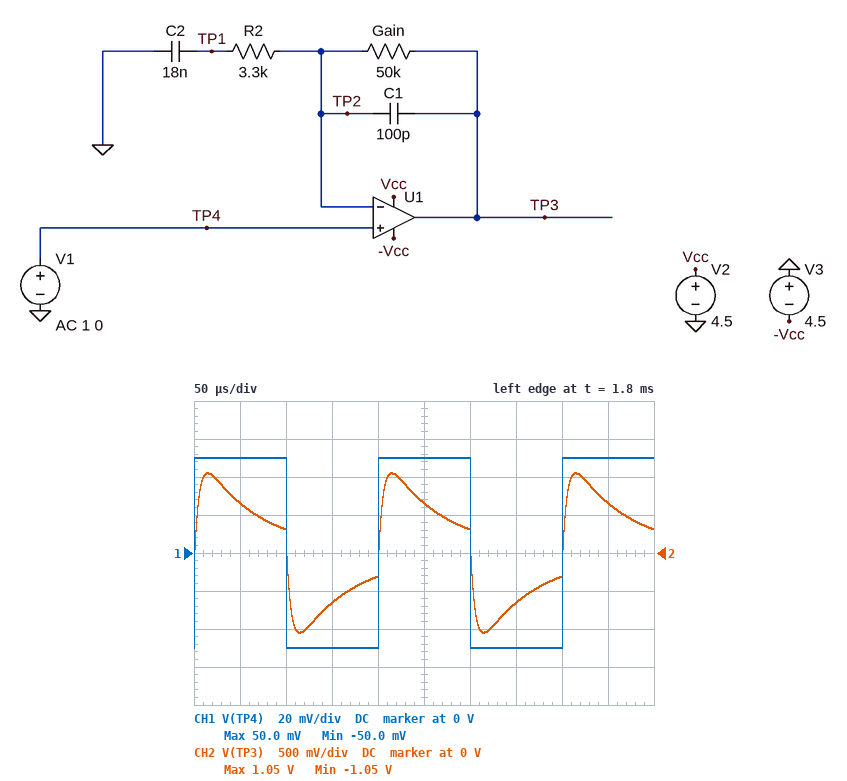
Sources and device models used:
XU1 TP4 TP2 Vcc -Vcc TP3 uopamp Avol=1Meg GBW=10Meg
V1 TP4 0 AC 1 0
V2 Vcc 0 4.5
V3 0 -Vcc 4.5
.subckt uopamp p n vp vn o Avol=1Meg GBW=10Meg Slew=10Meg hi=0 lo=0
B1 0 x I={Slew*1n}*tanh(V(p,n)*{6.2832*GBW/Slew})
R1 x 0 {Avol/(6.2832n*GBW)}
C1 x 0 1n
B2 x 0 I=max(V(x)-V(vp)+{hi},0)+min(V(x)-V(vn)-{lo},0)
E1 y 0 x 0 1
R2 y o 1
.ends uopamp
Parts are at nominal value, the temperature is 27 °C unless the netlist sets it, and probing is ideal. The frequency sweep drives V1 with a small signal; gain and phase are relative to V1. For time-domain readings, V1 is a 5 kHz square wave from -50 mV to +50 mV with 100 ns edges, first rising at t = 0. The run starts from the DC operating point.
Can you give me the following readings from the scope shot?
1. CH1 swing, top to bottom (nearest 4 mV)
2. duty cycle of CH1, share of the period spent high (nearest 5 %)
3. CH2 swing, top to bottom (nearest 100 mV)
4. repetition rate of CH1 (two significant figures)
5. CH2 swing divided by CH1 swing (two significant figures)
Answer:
100 mV
50 %
2.1 V
5.0 kHz
21
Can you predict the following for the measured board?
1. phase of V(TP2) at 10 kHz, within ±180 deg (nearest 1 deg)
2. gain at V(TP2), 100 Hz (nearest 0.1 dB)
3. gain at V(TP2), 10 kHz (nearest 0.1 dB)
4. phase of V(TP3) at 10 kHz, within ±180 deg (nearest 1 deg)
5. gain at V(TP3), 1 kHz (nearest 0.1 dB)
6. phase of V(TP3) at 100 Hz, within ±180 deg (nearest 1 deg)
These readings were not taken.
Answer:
-1 deg
0 dB
0 dB
-3 deg
15.2 dB
29 deg
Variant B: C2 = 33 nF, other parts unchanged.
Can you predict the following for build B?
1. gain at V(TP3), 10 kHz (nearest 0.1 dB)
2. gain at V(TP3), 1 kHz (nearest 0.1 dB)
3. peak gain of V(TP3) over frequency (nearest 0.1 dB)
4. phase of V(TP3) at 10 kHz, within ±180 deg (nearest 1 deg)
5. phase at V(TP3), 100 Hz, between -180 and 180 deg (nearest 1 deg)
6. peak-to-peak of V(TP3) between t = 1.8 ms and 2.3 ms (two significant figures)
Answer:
23.7 dB
19.3 dB
23.8 dB
-9 deg
44 deg
1.9 V
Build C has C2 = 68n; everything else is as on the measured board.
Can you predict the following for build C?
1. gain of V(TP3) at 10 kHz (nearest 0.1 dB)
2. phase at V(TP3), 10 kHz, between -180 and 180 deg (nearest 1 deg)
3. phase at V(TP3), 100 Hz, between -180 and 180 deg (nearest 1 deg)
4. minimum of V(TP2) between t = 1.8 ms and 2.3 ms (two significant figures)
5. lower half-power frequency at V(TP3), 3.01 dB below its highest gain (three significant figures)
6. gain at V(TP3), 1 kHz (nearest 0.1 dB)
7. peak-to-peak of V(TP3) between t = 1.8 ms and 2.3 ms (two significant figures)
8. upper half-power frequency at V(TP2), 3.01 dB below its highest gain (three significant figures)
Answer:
23.7 dB
-13 deg
58 deg
-50 mV
676 Hz
22.4 dB
1.8 V
9.47 MHz
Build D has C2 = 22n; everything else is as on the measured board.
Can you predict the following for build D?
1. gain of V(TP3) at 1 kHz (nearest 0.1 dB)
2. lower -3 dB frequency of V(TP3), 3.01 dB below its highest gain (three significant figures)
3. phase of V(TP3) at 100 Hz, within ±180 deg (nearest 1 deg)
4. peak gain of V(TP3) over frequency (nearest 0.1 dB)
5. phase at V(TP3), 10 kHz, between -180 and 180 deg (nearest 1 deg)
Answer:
16.6 dB
1.93 kHz
34 deg
23.6 dB
-6 deg
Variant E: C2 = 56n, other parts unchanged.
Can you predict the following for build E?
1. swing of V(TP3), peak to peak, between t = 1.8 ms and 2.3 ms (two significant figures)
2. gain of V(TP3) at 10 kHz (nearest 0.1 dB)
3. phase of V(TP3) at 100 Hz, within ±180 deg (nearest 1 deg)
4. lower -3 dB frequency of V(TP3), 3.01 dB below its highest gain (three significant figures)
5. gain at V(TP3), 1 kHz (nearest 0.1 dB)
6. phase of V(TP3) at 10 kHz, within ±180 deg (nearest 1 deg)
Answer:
1.8 V
23.7 dB
55 deg
814 Hz
21.8 dB
-13 deg
